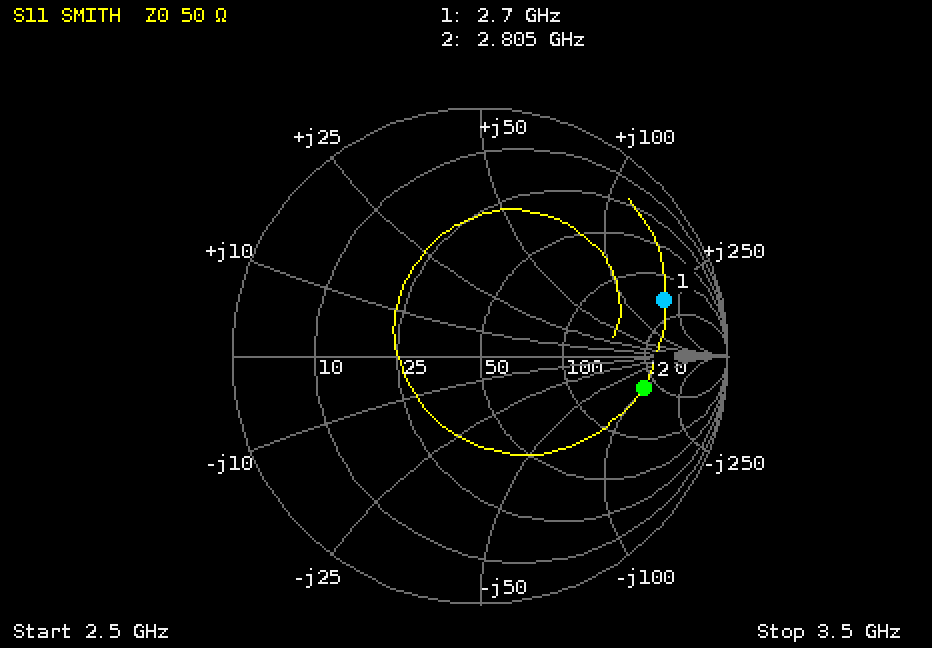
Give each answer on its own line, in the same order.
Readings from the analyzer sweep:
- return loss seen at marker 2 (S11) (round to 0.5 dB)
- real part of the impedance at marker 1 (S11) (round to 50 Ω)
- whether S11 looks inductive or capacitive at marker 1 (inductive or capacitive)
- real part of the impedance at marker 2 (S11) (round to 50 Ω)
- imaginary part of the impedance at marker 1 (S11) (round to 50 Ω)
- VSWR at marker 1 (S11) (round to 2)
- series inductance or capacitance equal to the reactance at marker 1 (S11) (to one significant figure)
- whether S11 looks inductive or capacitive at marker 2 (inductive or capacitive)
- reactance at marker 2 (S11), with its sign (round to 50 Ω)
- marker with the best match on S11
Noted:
3.5 dB
150 Ω
inductive
200 Ω
+200 Ω
8
10 nH
capacitive
-100 Ω
marker 2
